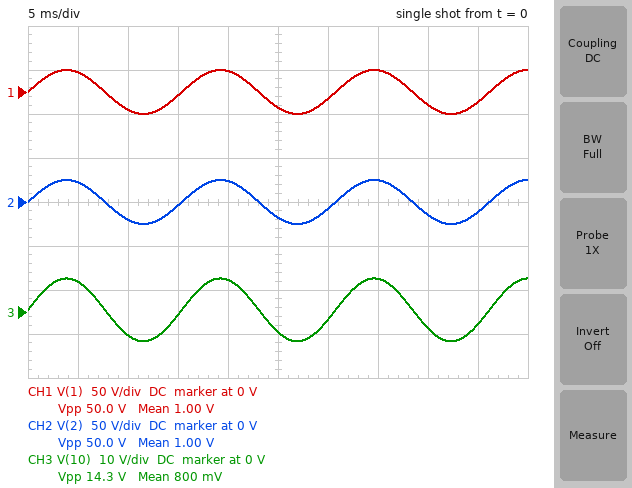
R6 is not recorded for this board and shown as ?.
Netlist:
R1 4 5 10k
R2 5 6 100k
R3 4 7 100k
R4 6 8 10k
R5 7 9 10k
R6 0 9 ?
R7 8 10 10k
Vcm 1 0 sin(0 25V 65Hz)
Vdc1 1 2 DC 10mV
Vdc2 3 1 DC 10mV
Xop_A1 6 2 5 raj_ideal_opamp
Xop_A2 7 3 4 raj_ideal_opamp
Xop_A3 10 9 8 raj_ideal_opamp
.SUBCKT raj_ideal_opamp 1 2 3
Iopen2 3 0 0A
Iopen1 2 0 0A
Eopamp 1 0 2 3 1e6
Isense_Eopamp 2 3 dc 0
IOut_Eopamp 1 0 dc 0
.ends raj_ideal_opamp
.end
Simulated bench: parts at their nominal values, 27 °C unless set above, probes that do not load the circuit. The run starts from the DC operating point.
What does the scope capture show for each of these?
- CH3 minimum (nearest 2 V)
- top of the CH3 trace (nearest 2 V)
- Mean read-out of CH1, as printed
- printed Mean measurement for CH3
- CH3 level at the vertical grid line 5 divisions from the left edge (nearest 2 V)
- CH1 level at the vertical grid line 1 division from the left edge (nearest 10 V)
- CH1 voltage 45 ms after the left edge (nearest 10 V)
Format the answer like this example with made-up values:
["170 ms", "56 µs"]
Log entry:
["-6 V", "8 V", "1.00 V", "800 mV", "-4 V", "20 V", "-10 V"]
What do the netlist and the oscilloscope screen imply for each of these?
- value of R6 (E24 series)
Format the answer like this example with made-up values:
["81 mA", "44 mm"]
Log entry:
["18 kΩ"]
